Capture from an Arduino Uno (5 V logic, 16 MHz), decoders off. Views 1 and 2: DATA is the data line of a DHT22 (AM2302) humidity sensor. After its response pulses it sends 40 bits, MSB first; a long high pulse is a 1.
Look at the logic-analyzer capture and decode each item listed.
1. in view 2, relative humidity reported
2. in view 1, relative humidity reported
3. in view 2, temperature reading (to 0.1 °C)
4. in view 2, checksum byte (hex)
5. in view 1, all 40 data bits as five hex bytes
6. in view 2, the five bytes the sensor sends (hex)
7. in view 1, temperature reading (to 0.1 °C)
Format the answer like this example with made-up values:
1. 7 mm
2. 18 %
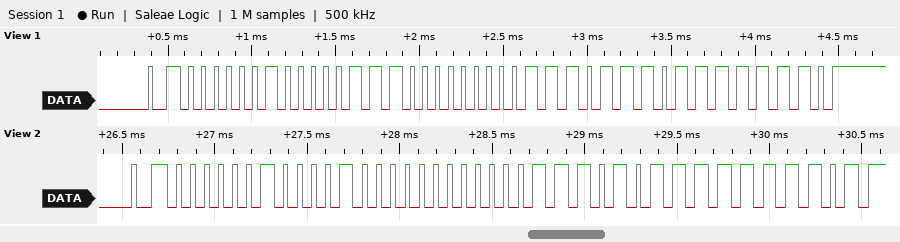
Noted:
1. 52.8 %
2. 52.6 %
3. 23.5 °C
4. 0xFD
5. 02 0E 00 EE FE
6. 02 10 00 EB FD
7. 23.8 °C
